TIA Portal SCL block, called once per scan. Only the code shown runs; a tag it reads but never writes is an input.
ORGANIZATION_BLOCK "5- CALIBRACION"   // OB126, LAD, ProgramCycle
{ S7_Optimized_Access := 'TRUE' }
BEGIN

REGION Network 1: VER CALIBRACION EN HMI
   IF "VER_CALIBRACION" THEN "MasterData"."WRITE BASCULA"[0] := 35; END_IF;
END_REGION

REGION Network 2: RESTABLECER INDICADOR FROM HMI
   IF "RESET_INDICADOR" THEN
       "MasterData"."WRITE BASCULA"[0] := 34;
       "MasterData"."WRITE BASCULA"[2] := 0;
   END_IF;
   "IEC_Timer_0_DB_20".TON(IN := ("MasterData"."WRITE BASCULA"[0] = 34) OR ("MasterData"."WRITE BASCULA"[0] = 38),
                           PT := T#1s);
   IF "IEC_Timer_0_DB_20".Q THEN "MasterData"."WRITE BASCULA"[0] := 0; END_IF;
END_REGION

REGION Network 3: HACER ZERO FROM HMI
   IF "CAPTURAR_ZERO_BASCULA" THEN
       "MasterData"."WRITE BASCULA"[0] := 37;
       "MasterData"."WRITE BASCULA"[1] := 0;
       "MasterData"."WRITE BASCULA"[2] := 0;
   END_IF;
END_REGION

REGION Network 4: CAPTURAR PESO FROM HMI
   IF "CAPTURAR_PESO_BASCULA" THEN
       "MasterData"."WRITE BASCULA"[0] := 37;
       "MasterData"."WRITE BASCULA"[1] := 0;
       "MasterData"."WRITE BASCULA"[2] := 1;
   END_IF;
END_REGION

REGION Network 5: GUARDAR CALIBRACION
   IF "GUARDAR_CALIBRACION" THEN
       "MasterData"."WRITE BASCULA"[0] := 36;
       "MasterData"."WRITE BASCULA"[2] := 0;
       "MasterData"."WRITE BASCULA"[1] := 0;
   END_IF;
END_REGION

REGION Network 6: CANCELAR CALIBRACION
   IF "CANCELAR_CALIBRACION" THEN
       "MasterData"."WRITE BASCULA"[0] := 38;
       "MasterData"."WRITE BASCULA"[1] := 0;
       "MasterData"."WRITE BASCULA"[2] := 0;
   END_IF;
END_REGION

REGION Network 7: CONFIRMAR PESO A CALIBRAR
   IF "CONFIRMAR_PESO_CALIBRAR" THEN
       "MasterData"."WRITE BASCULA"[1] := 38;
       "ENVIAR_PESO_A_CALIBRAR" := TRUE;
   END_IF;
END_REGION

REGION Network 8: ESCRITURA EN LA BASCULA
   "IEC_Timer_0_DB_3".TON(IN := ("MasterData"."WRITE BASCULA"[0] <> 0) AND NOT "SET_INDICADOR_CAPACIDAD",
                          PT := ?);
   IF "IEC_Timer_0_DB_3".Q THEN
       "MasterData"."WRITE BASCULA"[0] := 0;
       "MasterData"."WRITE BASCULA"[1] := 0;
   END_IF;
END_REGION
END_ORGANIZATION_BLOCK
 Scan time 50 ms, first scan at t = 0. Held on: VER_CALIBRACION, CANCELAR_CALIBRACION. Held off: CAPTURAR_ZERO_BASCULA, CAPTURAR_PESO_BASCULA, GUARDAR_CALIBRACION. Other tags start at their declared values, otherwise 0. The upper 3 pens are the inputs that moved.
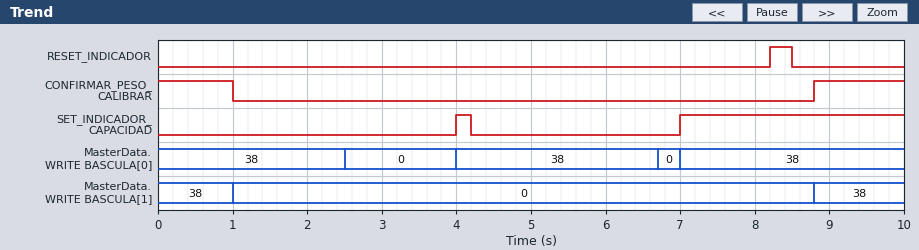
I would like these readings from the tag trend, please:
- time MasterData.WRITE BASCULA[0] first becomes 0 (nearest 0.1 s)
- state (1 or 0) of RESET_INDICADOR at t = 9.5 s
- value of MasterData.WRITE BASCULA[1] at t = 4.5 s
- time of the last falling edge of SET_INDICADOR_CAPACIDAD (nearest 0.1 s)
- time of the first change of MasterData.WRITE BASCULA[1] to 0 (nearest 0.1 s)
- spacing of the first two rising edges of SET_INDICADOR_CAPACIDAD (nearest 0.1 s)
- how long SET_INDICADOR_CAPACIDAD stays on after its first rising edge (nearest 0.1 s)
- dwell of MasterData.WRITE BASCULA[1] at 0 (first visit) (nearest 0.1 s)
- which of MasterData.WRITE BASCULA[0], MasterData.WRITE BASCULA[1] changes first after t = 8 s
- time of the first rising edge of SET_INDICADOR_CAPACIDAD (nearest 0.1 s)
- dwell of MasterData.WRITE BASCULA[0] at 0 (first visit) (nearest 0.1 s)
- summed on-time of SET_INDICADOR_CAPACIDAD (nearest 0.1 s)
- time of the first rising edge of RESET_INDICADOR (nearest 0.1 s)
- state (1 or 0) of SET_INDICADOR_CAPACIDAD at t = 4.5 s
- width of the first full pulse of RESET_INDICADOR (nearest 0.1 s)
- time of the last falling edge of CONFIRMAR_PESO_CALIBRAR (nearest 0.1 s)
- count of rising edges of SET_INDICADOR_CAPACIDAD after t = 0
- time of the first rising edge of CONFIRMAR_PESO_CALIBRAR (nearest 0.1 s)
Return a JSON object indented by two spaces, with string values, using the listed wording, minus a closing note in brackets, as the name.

{
  "time MasterData.WRITE BASCULA[0] first becomes 0": "2.5 s",
  "state (1 or 0) of RESET_INDICADOR at t = 9.5 s": "0",
  "value of MasterData.WRITE BASCULA[1] at t = 4.5 s": "0",
  "time of the last falling edge of SET_INDICADOR_CAPACIDAD": "4.2 s",
  "time of the first change of MasterData.WRITE BASCULA[1] to 0": "1.0 s",
  "spacing of the first two rising edges of SET_INDICADOR_CAPACIDAD": "3.0 s",
  "how long SET_INDICADOR_CAPACIDAD stays on after its first rising edge": "0.2 s",
  "dwell of MasterData.WRITE BASCULA[1] at 0 (first visit)": "7.8 s",
  "which of MasterData.WRITE BASCULA[0], MasterData.WRITE BASCULA[1] changes first after t = 8 s": "MasterData.WRITE BASCULA[1]",
  "time of the first rising edge of SET_INDICADOR_CAPACIDAD": "4.0 s",
  "dwell of MasterData.WRITE BASCULA[0] at 0 (first visit)": "1.5 s",
  "summed on-time of SET_INDICADOR_CAPACIDAD": "3.2 s",
  "time of the first rising edge of RESET_INDICADOR": "8.2 s",
  "state (1 or 0) of SET_INDICADOR_CAPACIDAD at t = 4.5 s": "0",
  "width of the first full pulse of RESET_INDICADOR": "0.3 s",
  "time of the last falling edge of CONFIRMAR_PESO_CALIBRAR": "1.0 s",
  "count of rising edges of SET_INDICADOR_CAPACIDAD after t = 0": "2",
  "time of the first rising edge of CONFIRMAR_PESO_CALIBRAR": "8.8 s"
}
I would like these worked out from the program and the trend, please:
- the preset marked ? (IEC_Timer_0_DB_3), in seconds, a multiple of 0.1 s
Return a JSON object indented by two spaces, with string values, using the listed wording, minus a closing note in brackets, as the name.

{
  "the preset marked ? (IEC_Timer_0_DB_3), in seconds, a multiple of 0.1 s": "2.5 s"
}
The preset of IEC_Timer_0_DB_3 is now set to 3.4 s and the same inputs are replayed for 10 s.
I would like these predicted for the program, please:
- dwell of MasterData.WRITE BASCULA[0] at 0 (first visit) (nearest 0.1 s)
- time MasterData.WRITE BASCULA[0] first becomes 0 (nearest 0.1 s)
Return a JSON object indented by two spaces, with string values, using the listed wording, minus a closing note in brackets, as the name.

{
  "dwell of MasterData.WRITE BASCULA[0] at 0 (first visit)": "0.6 s",
  "time MasterData.WRITE BASCULA[0] first becomes 0": "3.4 s"
}
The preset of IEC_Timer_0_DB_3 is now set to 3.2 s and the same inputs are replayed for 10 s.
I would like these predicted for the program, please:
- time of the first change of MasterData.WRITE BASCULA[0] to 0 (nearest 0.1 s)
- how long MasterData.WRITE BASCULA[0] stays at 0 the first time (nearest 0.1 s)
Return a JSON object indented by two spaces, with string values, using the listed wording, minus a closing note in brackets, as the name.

{
  "time of the first change of MasterData.WRITE BASCULA[0] to 0": "3.2 s",
  "how long MasterData.WRITE BASCULA[0] stays at 0 the first time": "0.8 s"
}
